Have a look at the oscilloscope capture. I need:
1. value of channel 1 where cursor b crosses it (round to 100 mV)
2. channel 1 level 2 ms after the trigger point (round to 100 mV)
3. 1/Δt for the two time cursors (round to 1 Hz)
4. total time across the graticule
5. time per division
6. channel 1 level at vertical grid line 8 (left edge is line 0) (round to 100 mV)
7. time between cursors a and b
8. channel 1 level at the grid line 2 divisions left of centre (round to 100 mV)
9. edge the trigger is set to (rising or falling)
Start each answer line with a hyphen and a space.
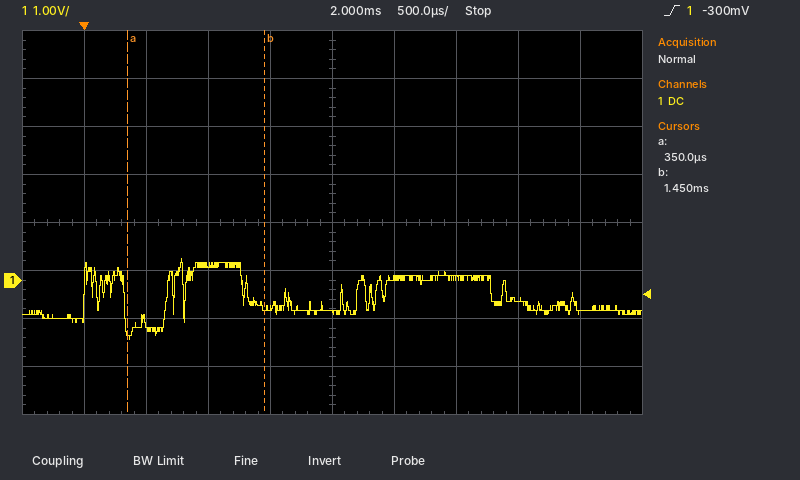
- -500 mV
- -700 mV
- 909 Hz
- 5 ms
- 500 µs
- -400 mV
- 1.10 ms
- 300 mV
- rising
